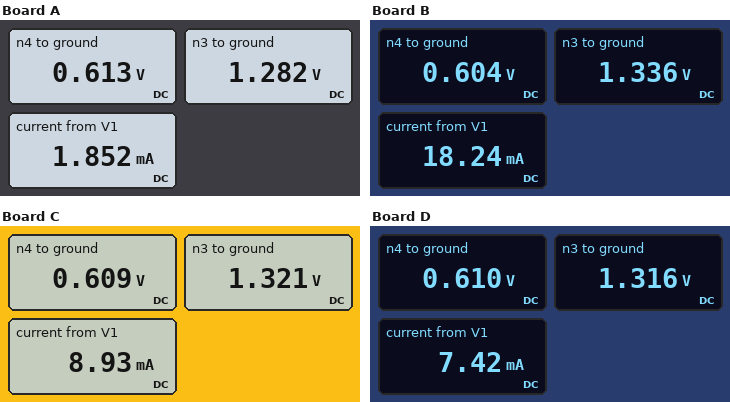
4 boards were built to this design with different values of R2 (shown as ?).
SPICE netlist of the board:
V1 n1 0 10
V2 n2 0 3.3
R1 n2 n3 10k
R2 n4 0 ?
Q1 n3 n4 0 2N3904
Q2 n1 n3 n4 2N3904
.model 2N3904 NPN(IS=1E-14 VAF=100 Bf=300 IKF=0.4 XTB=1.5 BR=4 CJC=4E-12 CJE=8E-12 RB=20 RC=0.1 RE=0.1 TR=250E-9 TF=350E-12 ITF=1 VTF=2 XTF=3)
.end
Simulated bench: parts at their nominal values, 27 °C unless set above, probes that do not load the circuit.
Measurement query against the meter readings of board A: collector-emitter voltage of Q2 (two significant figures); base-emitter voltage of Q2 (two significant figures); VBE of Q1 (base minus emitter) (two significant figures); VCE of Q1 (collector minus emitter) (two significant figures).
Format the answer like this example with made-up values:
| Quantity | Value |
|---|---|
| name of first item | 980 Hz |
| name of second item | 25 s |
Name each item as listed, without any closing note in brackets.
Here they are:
| Quantity | Value |
|---|---|
| collector-emitter voltage of Q2 | 9.4 V |
| base-emitter voltage of Q2 | 670 mV |
| VBE of Q1 (base minus emitter) | 610 mV |
| VCE of Q1 (collector minus emitter) | 1.3 V |
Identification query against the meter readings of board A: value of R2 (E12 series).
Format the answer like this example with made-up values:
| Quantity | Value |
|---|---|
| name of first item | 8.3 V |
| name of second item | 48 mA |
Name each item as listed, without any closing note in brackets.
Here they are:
| Quantity | Value |
|---|---|
| value of R2 | 330 Ω |
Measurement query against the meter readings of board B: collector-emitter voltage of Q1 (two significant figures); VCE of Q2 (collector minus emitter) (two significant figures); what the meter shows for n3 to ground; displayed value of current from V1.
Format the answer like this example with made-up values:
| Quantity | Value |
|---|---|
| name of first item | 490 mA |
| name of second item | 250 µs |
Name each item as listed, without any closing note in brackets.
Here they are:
| Quantity | Value |
|---|---|
| collector-emitter voltage of Q1 | 1.3 V |
| VCE of Q2 (collector minus emitter) | 9.4 V |
| what the meter shows for n3 to ground | 1.336 V |
| displayed value of current from V1 | 18.24 mA |
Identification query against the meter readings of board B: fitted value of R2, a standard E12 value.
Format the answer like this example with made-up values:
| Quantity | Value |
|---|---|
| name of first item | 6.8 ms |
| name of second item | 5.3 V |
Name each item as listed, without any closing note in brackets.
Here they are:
| Quantity | Value |
|---|---|
| fitted value of R2, a standard E12 value | 33 Ω |
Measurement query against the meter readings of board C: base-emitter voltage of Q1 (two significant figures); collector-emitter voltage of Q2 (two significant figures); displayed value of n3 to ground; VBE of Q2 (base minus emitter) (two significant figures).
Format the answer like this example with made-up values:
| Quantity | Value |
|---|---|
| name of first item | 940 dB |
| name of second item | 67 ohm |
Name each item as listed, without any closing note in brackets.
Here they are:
| Quantity | Value |
|---|---|
| base-emitter voltage of Q1 | 610 mV |
| collector-emitter voltage of Q2 | 9.4 V |
| displayed value of n3 to ground | 1.321 V |
| VBE of Q2 (base minus emitter) | 710 mV |
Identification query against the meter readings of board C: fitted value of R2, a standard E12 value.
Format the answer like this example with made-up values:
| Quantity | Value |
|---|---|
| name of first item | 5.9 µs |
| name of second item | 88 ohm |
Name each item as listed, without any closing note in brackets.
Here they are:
| Quantity | Value |
|---|---|
| fitted value of R2, a standard E12 value | 68 Ω |
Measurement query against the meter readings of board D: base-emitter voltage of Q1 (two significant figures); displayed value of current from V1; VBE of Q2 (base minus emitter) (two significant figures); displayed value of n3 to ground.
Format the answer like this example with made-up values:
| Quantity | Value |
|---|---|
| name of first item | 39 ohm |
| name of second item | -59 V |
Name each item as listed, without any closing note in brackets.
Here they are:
| Quantity | Value |
|---|---|
| base-emitter voltage of Q1 | 610 mV |
| displayed value of current from V1 | 7.42 mA |
| VBE of Q2 (base minus emitter) | 710 mV |
| displayed value of n3 to ground | 1.316 V |
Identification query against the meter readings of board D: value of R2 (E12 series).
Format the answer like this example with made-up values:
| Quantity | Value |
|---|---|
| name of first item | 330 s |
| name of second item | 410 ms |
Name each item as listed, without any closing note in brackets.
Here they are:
| Quantity | Value |
|---|---|
| value of R2 | 82 Ω |
